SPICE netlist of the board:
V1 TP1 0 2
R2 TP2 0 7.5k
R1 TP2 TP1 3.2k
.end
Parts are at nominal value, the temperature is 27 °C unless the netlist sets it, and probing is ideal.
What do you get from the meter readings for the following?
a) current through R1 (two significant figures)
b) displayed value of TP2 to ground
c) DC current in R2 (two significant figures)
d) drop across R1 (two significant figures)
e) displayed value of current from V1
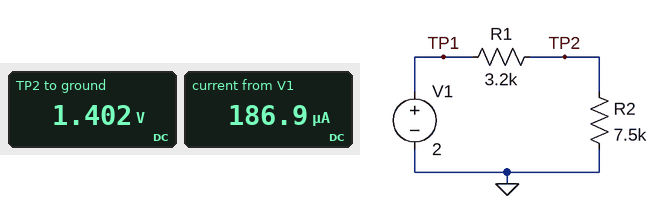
190 µA
1.402 V
190 µA
600 mV
186.9 µA
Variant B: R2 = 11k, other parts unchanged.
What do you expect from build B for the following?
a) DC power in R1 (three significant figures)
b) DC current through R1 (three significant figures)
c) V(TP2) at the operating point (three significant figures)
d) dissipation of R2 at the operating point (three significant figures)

63.5 µW
141 µA
1.55 V
218 µW
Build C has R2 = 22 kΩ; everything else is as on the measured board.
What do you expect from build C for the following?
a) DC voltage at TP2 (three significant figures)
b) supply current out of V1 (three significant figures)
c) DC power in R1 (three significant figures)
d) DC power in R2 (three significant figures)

1.75 V
79.4 µA
20.2 µW
139 µW
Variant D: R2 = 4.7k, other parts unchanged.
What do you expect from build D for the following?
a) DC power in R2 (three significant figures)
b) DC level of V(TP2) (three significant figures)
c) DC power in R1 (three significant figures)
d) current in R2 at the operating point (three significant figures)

301 µW
1.19 V
205 µW
253 µA
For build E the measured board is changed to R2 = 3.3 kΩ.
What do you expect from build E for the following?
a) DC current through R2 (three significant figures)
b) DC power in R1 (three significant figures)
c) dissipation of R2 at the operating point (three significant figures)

308 µA
303 µW
312 µW
